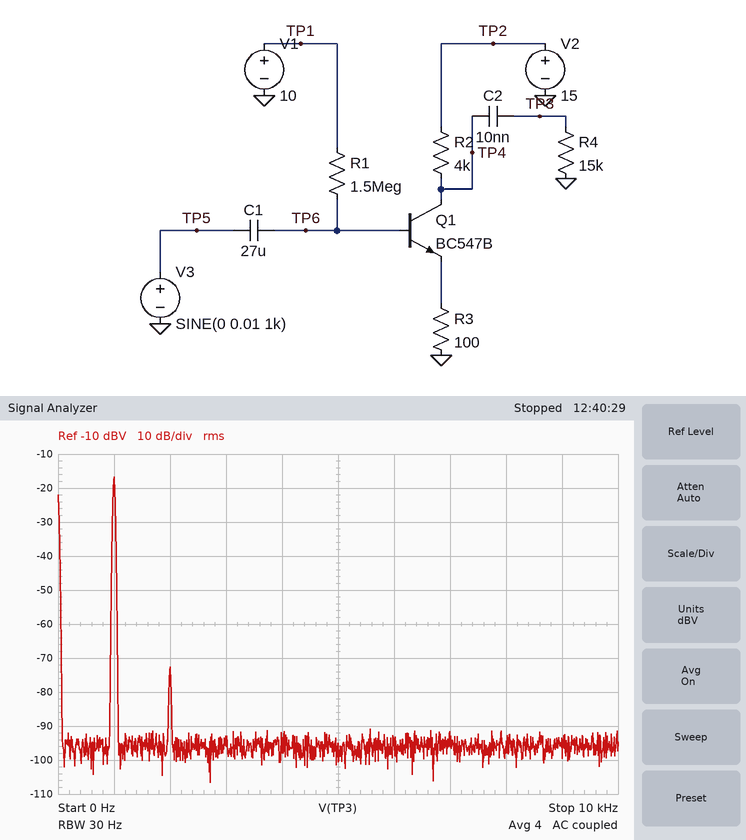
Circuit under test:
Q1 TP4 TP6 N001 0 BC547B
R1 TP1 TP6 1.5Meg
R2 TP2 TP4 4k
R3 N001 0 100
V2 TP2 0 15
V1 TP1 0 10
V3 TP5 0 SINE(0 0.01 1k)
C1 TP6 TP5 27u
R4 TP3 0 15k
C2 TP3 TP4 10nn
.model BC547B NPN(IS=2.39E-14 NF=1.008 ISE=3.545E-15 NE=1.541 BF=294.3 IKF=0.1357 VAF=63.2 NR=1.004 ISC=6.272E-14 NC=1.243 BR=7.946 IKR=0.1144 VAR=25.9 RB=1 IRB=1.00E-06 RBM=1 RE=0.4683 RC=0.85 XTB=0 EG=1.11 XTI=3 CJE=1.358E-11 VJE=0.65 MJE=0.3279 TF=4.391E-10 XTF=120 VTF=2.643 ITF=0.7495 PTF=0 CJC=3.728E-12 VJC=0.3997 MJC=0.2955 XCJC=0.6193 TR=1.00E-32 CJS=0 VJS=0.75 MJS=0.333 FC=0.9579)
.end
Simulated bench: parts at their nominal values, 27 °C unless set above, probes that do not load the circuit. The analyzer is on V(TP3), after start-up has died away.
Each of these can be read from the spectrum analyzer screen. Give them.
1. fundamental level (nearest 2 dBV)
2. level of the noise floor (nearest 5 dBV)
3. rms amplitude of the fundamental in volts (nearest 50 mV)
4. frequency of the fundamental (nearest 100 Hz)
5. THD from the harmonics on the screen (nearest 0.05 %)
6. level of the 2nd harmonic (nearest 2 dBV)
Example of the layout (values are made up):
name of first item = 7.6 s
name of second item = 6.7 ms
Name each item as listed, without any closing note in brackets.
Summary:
fundamental level = -16 dBV
level of the noise floor = -95 dBV
rms amplitude of the fundamental in volts = 150 mV
frequency of the fundamental = 1.0 kHz
THD from the harmonics on the screen = 0.15 %
level of the 2nd harmonic = -72 dBV
